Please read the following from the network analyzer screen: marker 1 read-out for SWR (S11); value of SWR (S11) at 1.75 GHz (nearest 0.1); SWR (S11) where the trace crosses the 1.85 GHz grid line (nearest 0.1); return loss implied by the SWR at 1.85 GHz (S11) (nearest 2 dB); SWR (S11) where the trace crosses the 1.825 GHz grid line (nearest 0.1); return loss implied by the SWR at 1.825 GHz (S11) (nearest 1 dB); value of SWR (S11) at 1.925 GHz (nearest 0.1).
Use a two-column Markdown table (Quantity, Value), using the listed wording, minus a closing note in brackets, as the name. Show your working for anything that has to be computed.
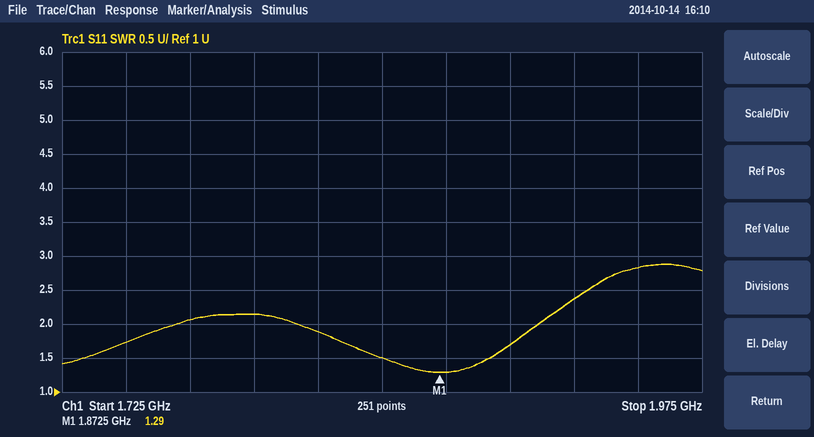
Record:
| Quantity | Value |
|---|---|
| marker 1 read-out for SWR | 1.29 |
| value of SWR (S11) at 1.75 GHz | 1.7 |
| SWR (S11) where the trace crosses the 1.85 GHz grid line | 1.5 |
| return loss implied by the SWR at 1.85 GHz (S11) | −20 log10((1.5 − 1)/(1.5 + 1)) ≈ 14 dB |
| SWR (S11) where the trace crosses the 1.825 GHz grid line | 1.9 |
| return loss implied by the SWR at 1.825 GHz (S11) | −20 log10((1.9 − 1)/(1.9 + 1)) ≈ 10 dB |
| value of SWR (S11) at 1.925 GHz | 2.4 |
